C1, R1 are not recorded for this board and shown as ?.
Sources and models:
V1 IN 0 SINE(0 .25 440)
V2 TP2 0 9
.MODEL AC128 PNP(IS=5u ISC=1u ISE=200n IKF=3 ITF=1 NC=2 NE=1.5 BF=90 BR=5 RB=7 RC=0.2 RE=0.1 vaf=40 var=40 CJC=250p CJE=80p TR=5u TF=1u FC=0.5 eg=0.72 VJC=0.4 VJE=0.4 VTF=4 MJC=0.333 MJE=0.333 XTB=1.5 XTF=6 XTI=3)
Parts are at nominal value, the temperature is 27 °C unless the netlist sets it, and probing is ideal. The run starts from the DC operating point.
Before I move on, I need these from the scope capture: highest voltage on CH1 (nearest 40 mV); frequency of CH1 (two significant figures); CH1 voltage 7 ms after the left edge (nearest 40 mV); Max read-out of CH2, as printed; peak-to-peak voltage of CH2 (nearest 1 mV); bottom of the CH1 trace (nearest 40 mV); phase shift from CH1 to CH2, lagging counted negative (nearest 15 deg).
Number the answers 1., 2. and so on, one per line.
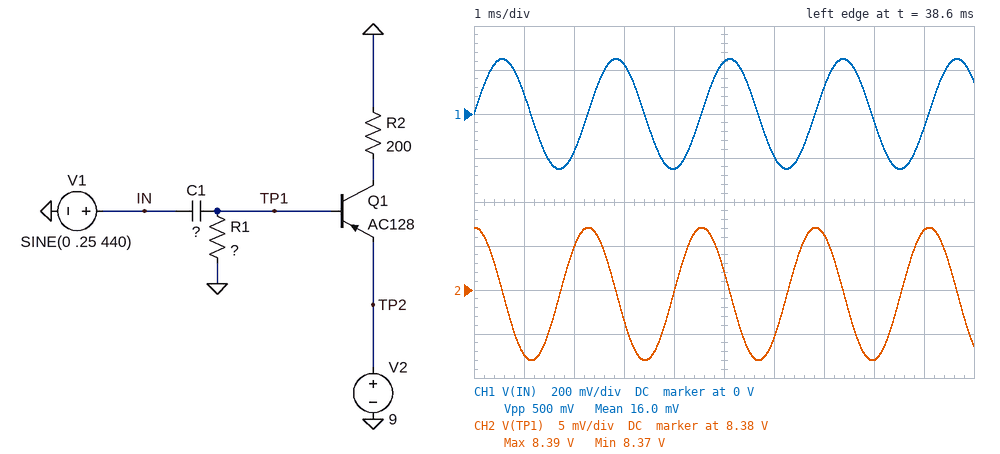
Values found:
1. 240 mV
2. 440 Hz
3. 120 mV
4. 8.39 V
5. 15 mV
6. -240 mV
7. 90 deg
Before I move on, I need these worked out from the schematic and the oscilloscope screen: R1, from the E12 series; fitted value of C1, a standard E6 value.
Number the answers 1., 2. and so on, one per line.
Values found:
1. 180 Ω
2. 1.5 µF
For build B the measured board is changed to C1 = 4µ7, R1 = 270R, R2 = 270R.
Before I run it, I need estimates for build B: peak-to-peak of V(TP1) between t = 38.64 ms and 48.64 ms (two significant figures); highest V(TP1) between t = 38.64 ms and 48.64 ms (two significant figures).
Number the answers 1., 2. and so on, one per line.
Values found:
1. 49 mV
2. 8.5 V
